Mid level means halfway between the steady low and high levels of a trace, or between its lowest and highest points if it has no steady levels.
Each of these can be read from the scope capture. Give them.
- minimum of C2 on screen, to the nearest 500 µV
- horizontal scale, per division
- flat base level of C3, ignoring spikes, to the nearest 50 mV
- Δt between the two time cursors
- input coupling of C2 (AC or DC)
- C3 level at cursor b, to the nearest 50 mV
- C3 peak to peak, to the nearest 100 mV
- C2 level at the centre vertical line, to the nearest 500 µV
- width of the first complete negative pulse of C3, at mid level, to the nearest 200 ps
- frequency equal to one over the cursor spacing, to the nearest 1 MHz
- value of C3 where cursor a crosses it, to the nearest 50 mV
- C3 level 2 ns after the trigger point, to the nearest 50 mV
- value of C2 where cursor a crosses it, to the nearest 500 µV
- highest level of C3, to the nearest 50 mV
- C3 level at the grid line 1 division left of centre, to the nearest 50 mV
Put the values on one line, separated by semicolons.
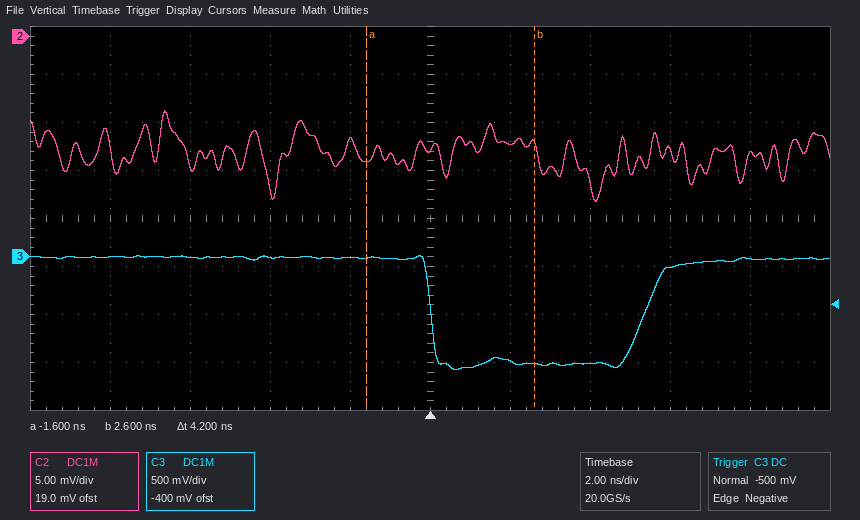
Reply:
-17.0 mV; 2 ns; -1.10 V; 4.2 ns; DC; -1.10 V; 1.20 V; -11.5 mV; 5.4 ns; 238 MHz; 0 mV; -1.10 V; -13.0 mV; 0 mV; 0 mV
